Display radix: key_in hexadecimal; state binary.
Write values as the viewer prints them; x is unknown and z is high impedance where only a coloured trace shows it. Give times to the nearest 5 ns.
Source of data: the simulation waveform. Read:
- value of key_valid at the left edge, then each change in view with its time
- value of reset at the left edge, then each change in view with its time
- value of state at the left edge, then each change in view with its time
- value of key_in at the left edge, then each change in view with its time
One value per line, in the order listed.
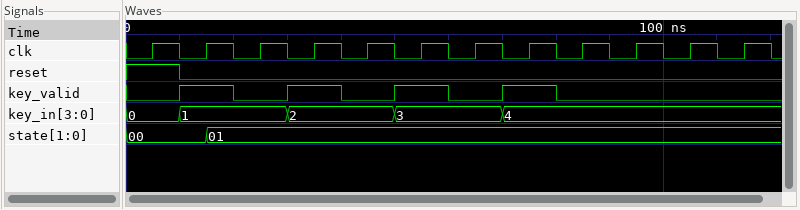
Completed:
0, 1 at 10 ns, 0 at 20 ns, 1 at 30 ns, 0 at 40 ns, 1 at 50 ns, 0 at 60 ns, 1 at 70 ns, 0 at 80 ns
1, 0 at 10 ns
00, 01 at 15 ns
0, 1 at 10 ns, 2 at 30 ns, 3 at 50 ns, 4 at 70 ns
